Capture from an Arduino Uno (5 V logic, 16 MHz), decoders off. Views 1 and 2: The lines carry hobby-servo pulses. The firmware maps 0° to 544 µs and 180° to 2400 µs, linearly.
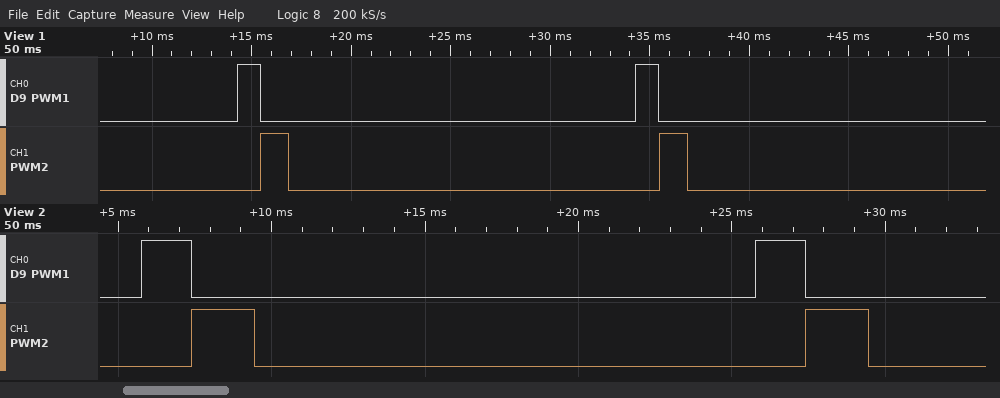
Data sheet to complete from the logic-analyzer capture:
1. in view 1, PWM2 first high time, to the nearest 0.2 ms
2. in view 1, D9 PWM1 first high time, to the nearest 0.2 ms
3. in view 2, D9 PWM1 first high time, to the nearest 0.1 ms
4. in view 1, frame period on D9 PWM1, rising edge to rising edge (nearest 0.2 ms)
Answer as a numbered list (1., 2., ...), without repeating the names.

1. 1.4 ms
2. 1.2 ms
3. 1.6 ms
4. 20.0 ms
